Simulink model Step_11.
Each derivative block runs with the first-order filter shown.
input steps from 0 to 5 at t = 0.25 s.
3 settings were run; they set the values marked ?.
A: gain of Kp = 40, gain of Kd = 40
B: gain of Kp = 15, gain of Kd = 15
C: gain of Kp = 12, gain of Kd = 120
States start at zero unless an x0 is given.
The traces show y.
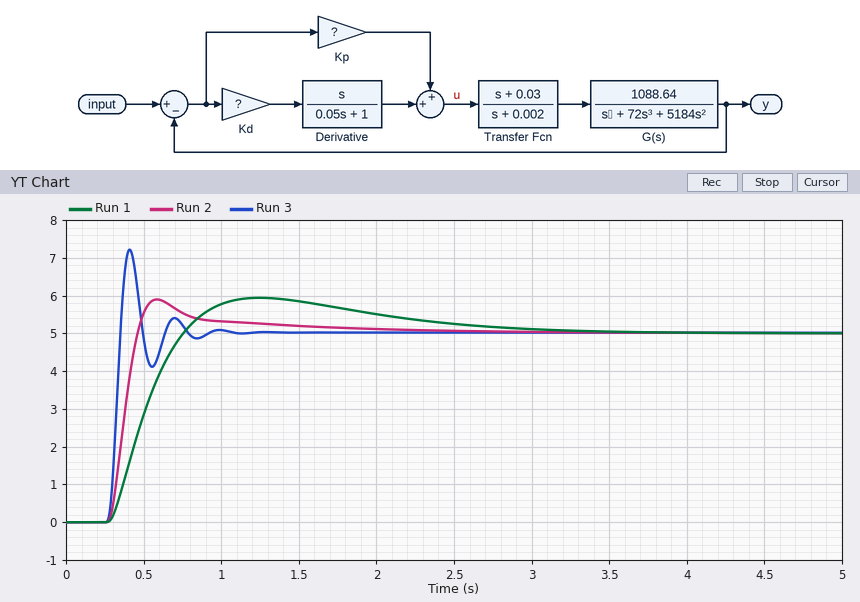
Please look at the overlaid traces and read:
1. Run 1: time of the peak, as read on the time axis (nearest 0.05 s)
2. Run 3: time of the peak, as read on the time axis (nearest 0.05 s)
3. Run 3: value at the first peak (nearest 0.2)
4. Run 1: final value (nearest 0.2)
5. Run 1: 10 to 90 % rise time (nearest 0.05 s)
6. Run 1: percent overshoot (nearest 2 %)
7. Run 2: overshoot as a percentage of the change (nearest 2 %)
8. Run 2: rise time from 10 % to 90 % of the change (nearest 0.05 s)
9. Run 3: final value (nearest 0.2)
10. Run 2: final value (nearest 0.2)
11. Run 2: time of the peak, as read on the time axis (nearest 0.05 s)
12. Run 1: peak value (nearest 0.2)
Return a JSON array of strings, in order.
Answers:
["1.25 s", "0.40 s", "7.2", "5.0", "0.35 s", "18 %", "18 %", "0.15 s", "5.0", "5.0", "0.60 s", "6.0"]
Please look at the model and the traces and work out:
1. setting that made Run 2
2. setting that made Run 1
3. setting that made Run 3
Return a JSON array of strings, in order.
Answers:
["A", "B", "C"]
